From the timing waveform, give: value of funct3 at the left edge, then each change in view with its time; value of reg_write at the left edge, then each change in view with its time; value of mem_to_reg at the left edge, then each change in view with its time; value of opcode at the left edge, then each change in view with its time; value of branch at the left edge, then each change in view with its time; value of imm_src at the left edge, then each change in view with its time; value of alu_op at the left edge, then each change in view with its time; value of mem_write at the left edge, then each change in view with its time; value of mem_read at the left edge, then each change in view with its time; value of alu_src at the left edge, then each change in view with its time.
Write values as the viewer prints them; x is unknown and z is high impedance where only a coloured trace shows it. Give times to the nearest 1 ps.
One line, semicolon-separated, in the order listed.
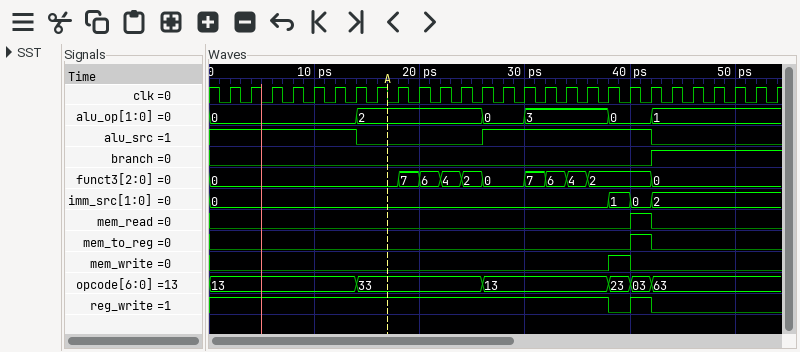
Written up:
0, 7 at 18 ps, 6 at 20 ps, 4 at 22 ps, 2 at 24 ps, 0 at 26 ps, 7 at 30 ps, 6 at 32 ps, 4 at 34 ps, 2 at 36 ps, 0 at 42 ps; 1, 0 at 38 ps, 1 at 40 ps, 0 at 42 ps; 0, 1 at 40 ps, 0 at 42 ps; 13, 33 at 14 ps, 13 at 26 ps, 23 at 38 ps, 03 at 40 ps, 63 at 42 ps; 0, 1 at 42 ps; 0, 1 at 38 ps, 0 at 40 ps, 2 at 42 ps; 0, 2 at 14 ps, 0 at 26 ps, 3 at 30 ps, 0 at 38 ps, 1 at 42 ps; 0, 1 at 38 ps, 0 at 40 ps; 0, 1 at 40 ps, 0 at 42 ps; 1, 0 at 14 ps, 1 at 26 ps, 0 at 42 ps
